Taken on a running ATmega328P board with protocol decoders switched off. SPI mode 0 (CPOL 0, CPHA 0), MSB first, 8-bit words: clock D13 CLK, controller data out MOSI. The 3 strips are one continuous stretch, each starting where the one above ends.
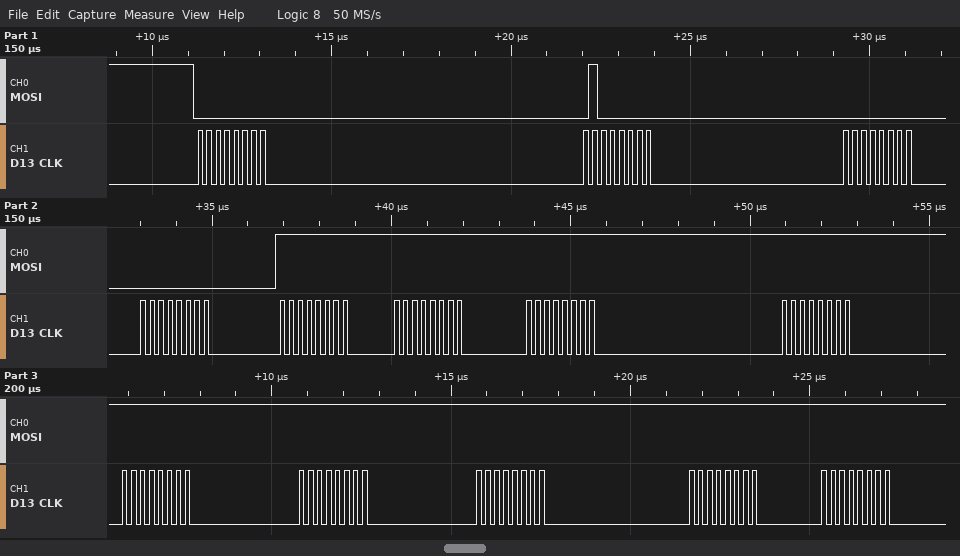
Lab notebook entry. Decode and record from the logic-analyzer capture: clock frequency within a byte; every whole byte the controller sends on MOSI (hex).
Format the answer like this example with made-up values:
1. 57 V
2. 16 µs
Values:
1. 4 MHz
2. 0x00 0x40 0x00 0x00 0xFF 0xFF 0xFF 0xFF 0xFF 0xFF 0xFF 0xFF 0xFF
